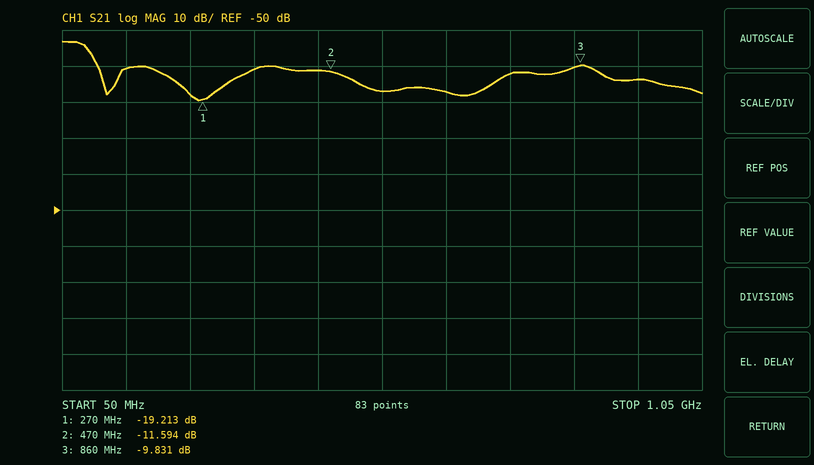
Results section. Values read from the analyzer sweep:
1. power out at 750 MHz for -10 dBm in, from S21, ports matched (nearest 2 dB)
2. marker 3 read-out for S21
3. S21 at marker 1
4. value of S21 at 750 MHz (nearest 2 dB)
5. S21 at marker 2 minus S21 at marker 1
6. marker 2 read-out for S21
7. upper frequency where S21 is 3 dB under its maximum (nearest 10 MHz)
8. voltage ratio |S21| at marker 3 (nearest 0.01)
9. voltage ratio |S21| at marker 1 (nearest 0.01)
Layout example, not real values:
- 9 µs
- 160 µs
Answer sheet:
- -22 dBm
- -9.831 dB
- -19.213 dB
- -12 dB
- 7.619 dB
- -11.594 dB
- 90 MHz
- 0.32
- 0.11
